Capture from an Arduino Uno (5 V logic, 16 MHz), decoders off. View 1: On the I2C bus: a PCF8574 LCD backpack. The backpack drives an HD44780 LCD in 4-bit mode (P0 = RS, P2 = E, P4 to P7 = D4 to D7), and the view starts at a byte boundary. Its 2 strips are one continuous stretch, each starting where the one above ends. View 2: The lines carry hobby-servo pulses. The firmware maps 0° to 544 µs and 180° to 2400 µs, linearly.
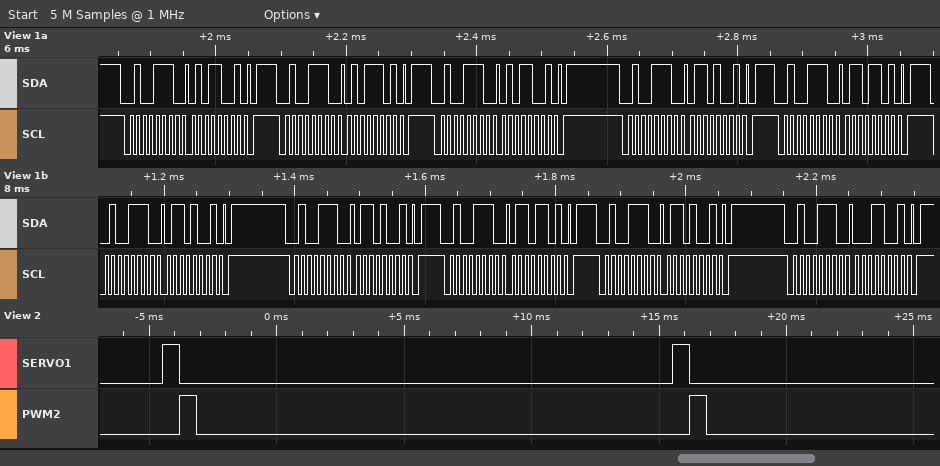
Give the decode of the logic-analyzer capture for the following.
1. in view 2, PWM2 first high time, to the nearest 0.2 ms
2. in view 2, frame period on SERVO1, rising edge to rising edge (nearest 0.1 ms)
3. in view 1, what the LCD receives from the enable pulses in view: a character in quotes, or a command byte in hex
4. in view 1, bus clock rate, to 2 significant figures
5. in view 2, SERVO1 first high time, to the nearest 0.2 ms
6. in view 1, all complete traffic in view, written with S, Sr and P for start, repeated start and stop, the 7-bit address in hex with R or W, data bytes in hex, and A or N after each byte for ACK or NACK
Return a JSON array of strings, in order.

["0.6 ms", "20.0 ms", "'V'", "100 kHz", "0.6 ms", "S 27W A 59 A P S 27W A 5D A P S 27W A 59 A P S 27W A 69 A P S 27W A 6D A P S 27W A 69 A P S 27W A 69 A P S 27W A 6D A P S 27W A 69 A P S 27W A 19 A P"]
